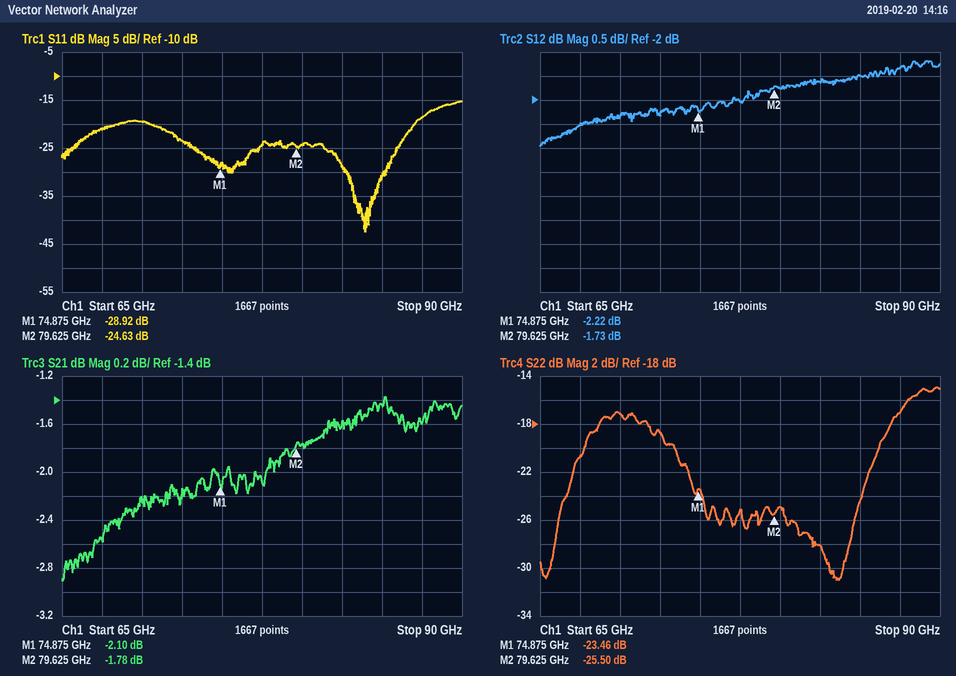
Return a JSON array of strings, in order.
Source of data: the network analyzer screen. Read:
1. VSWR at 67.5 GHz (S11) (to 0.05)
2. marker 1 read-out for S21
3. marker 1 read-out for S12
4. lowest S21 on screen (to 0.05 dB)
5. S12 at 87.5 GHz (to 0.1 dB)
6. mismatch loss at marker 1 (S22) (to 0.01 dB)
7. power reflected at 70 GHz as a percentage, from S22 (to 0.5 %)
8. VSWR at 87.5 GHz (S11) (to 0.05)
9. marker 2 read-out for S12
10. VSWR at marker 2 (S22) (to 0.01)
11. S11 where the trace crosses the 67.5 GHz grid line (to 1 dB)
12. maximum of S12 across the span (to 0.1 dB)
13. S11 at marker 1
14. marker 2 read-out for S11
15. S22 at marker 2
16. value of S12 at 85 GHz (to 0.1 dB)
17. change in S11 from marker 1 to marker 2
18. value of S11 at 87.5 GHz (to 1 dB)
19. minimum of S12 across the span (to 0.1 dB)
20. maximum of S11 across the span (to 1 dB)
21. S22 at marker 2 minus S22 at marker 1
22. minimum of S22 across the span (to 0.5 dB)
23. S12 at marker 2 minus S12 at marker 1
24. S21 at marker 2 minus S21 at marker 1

["1.20", "-2.10 dB", "-2.22 dB", "-2.90 dB", "-1.3 dB", "0.02 dB", "2.0 %", "1.25", "-1.73 dB", "1.11", "-21 dB", "-1.2 dB", "-28.92 dB", "-24.63 dB", "-25.50 dB", "-1.5 dB", "4.29 dB", "-19 dB", "-3.0 dB", "-15 dB", "-2.04 dB", "-31.0 dB", "0.49 dB", "0.32 dB"]
